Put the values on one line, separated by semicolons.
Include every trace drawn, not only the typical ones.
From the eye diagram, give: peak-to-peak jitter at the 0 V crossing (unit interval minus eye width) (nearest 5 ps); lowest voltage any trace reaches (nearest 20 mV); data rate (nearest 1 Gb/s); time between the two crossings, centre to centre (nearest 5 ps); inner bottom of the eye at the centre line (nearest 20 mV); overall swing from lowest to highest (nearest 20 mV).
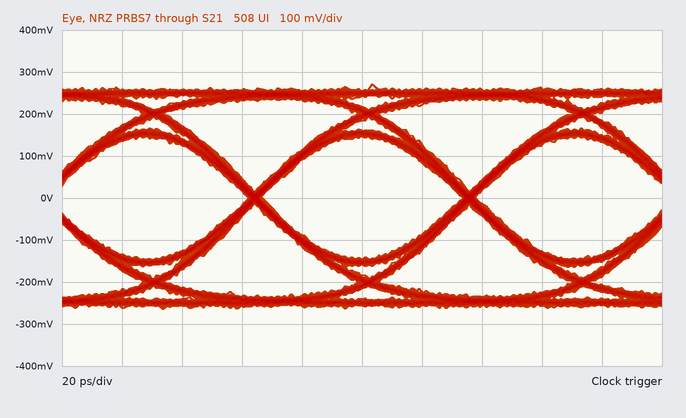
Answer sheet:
5 ps; -260 mV; 14 Gb/s; 70 ps; -140 mV; 540 mV
